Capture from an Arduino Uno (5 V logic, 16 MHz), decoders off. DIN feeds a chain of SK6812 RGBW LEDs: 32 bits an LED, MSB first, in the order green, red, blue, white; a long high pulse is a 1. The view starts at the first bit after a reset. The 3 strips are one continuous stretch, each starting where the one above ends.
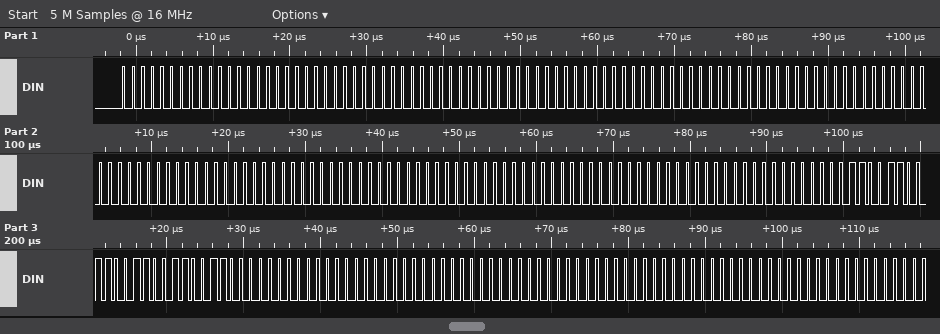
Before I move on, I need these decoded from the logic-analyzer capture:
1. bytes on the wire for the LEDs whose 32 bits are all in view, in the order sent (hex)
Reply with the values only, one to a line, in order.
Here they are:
00 00 00 00 00 00 00 00 00 00 00 00 00 00 00 00 00 00 00 00 33 33 33 00 00 00 00 00 00 00 00 00
